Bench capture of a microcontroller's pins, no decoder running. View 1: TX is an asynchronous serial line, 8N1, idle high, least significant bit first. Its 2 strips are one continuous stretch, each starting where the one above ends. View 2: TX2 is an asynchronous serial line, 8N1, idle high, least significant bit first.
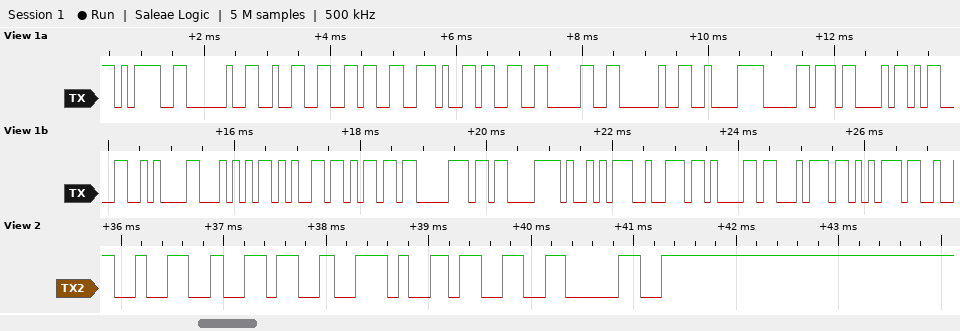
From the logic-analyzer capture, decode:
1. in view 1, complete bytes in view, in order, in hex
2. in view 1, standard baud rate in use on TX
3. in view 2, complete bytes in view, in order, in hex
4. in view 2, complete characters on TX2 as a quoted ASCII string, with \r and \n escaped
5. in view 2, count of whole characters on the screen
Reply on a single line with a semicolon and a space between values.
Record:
0x3D 0x20 0x32 0x36 0x2E 0x33 0x30 0x20 0xC2 0xB0 0x43 0x0D 0x0A 0x54 0x65 0x6D 0x70 0xC3 0xA9 0x72 0x61 0x74 0x75; 9600 baud; 32 36 2E 33 30; "26.30"; 5
